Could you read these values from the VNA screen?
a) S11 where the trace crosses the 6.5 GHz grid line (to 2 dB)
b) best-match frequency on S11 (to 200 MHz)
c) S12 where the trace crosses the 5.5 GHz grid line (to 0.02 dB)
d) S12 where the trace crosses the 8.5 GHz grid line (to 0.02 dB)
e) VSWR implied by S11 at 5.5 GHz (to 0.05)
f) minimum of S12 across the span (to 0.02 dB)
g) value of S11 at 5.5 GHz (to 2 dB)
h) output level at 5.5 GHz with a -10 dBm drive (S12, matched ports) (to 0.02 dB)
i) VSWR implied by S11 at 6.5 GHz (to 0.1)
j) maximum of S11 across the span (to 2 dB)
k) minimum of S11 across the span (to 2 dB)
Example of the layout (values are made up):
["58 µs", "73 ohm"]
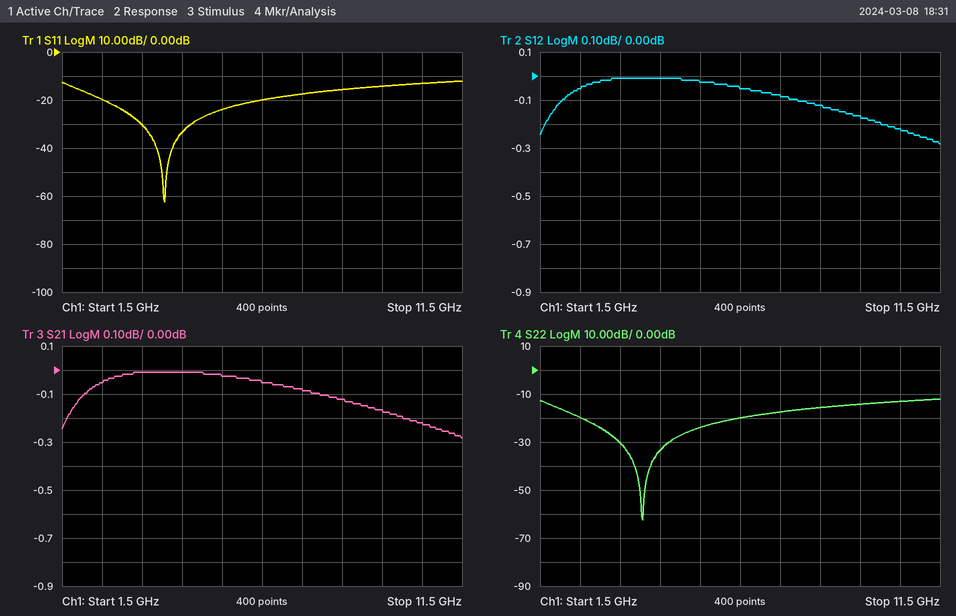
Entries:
["-20 dB", "4.0 GHz", "-0.02 dB", "-0.12 dB", "1.15", "-0.28 dB", "-24 dB", "-10.02 dBm", "1.2", "-12 dB", "-62 dB"]
